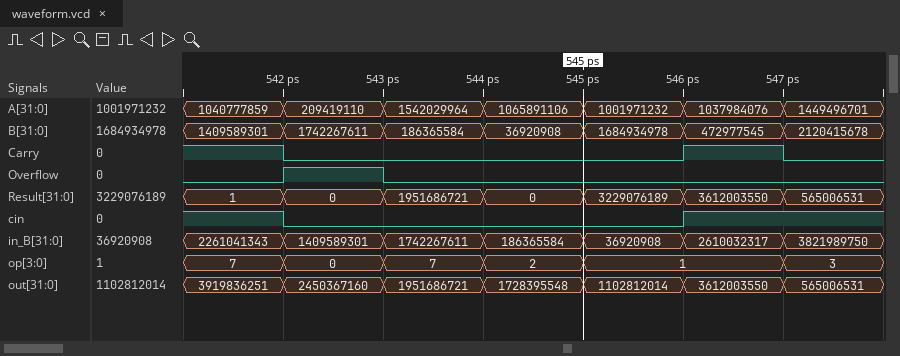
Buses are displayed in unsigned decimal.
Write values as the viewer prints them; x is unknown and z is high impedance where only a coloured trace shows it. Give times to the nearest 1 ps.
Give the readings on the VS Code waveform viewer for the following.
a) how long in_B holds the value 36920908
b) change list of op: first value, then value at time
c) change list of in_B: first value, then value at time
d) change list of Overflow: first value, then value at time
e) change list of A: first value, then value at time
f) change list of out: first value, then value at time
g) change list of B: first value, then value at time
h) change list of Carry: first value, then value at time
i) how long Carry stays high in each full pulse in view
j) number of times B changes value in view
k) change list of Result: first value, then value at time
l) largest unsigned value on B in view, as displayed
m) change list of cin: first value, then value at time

1 ps
7, 0 at 542 ps, 7 at 543 ps, 2 at 544 ps, 1 at 545 ps, 3 at 547 ps
2261041343, 1409589301 at 542 ps, 1742267611 at 543 ps, 186365584 at 544 ps, 36920908 at 545 ps, 2610032317 at 546 ps, 3821989750 at 547 ps
0, 1 at 542 ps, 0 at 543 ps
1040777859, 209419110 at 542 ps, 1542029964 at 543 ps, 1065891106 at 544 ps, 1001971232 at 545 ps, 1037984076 at 546 ps, 1449496701 at 547 ps
3919836251, 2450367160 at 542 ps, 1951686721 at 543 ps, 1728395548 at 544 ps, 1102812014 at 545 ps, 3612003550 at 546 ps, 565006531 at 547 ps
1409589301, 1742267611 at 542 ps, 186365584 at 543 ps, 36920908 at 544 ps, 1684934978 at 545 ps, 472977545 at 546 ps, 2120415678 at 547 ps
1, 0 at 542 ps, 1 at 546 ps, 0 at 547 ps
1 ps
6
1, 0 at 542 ps, 1951686721 at 543 ps, 0 at 544 ps, 3229076189 at 545 ps, 3612003550 at 546 ps, 565006531 at 547 ps
2120415678
1, 0 at 542 ps, 1 at 546 ps
